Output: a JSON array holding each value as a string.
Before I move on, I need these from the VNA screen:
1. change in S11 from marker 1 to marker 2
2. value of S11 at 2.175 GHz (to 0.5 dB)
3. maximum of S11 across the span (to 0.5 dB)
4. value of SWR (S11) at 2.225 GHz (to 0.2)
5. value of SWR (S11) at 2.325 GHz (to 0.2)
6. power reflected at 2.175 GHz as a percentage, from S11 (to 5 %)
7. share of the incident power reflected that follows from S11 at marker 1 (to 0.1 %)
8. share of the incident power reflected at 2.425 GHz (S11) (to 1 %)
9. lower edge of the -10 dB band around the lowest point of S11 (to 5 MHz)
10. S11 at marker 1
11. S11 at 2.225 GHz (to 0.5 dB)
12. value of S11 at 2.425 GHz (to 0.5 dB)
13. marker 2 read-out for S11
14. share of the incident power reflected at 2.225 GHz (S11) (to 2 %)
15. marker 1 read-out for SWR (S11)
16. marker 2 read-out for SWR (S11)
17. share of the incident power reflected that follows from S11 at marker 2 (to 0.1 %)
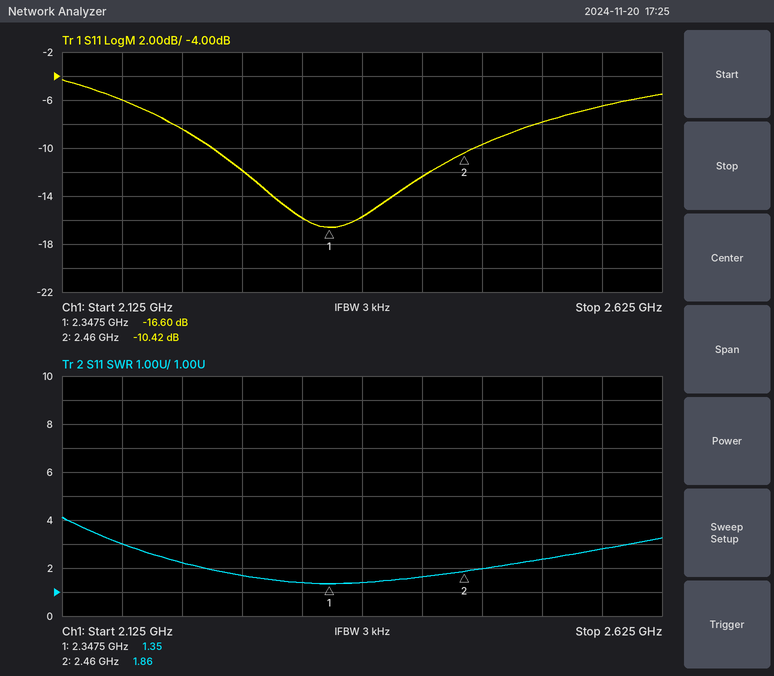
["6.18 dB", "-6.0 dB", "-4.5 dB", "2.2", "1.4", "25 %", "2.2 %", "6 %", "2.250 GHz", "-16.60 dB", "-8.5 dB", "-12.5 dB", "-10.42 dB", "14 %", "1.35", "1.86", "9.1 %"]
